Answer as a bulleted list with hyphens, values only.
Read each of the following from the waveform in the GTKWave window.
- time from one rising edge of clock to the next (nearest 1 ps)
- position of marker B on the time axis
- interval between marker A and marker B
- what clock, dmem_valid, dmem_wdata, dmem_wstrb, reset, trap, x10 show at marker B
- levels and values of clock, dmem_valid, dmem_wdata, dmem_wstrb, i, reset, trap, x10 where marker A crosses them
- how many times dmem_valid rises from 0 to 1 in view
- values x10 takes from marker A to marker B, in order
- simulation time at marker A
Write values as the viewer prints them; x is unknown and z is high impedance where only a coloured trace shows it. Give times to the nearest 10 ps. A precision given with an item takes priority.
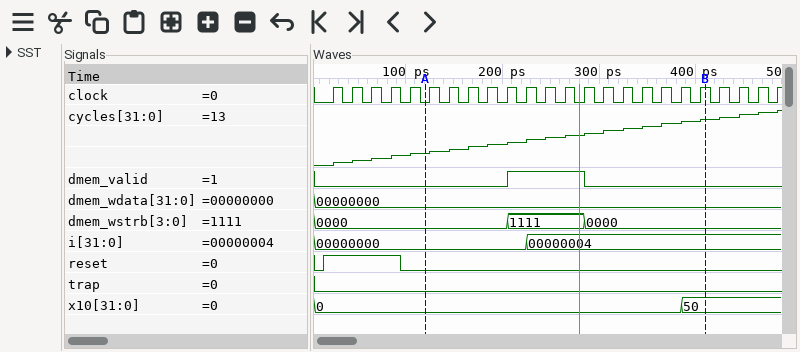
- 20 ps
- 410 ps
- 290 ps
- clock=1, dmem_valid=0, dmem_wdata=00000000, dmem_wstrb=0000, reset=0, trap=0, x10=50
- clock=0, dmem_valid=0, dmem_wdata=00000000, dmem_wstrb=0000, i=00000000, reset=0, trap=0, x10=0
- 1
- 0, 50
- 120 ps
